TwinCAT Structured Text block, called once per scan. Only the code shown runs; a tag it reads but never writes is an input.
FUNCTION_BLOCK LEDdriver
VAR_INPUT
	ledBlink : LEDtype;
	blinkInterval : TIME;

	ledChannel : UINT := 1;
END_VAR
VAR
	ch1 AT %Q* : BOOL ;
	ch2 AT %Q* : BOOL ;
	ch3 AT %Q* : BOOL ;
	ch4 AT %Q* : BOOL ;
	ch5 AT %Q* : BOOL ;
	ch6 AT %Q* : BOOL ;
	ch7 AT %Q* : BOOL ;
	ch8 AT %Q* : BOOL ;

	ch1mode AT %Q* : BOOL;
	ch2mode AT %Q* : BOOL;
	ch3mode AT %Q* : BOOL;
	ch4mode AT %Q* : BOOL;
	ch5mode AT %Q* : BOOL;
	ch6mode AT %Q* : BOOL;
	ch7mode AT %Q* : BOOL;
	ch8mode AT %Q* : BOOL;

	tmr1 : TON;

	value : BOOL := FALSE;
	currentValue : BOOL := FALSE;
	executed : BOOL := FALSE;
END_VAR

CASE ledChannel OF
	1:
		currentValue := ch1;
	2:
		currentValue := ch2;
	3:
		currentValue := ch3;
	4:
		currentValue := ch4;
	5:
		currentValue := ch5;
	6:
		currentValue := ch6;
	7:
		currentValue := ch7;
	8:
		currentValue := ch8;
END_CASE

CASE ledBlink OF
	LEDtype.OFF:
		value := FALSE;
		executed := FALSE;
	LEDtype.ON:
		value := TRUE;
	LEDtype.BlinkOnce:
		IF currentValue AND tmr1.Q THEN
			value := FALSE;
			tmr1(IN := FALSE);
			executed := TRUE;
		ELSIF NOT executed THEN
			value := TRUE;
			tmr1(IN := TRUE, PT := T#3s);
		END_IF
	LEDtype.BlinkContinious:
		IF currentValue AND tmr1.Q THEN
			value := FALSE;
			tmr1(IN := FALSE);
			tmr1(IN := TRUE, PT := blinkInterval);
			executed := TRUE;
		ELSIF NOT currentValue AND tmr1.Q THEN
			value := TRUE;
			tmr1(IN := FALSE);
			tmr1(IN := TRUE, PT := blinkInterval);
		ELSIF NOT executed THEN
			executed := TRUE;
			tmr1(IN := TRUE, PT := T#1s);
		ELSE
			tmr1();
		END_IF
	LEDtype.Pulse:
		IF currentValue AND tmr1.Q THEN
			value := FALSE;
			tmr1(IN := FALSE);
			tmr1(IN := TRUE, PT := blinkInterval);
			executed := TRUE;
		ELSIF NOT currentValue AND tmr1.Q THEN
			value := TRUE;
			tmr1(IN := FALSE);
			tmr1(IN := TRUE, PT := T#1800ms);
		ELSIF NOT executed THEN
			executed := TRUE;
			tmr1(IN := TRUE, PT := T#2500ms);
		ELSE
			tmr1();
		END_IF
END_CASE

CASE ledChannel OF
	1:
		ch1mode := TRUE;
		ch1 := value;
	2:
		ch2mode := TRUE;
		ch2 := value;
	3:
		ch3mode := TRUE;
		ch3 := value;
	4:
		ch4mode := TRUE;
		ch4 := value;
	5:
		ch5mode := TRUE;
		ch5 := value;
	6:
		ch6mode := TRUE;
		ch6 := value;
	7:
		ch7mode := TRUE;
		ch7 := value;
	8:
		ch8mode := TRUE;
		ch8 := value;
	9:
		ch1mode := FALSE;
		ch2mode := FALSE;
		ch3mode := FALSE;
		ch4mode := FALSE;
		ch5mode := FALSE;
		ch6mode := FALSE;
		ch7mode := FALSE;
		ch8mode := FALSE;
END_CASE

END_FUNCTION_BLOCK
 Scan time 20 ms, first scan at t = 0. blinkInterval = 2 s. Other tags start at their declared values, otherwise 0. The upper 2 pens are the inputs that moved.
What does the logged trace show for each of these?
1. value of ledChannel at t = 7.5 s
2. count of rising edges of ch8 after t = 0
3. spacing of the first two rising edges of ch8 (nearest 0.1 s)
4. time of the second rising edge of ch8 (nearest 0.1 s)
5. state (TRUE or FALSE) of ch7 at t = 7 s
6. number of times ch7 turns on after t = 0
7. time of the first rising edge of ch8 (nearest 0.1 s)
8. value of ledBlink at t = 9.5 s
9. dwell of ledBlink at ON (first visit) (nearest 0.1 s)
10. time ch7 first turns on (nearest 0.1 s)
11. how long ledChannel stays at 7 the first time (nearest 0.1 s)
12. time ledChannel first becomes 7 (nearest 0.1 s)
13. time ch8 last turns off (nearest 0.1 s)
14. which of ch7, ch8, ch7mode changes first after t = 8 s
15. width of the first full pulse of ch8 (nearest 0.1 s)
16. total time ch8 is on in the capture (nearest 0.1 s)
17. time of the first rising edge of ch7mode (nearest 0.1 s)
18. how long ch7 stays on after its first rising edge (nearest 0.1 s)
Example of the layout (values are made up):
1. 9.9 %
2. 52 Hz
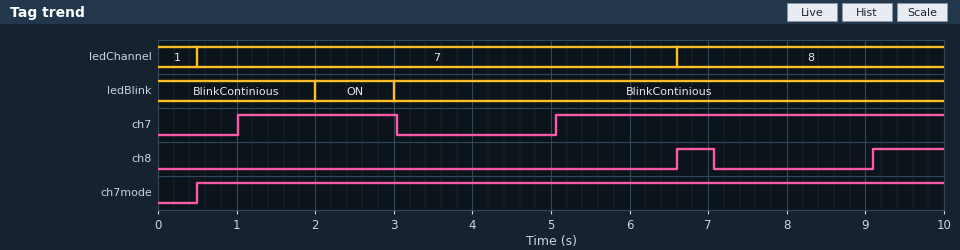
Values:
1. 8
2. 2
3. 2.5 s
4. 9.1 s
5. TRUE
6. 2
7. 6.6 s
8. BlinkContinious
9. 1.0 s
10. 1.0 s
11. 6.1 s
12. 0.5 s
13. 7.1 s
14. ch8
15. 0.5 s
16. 1.4 s
17. 0.5 s
18. 2.0 s
